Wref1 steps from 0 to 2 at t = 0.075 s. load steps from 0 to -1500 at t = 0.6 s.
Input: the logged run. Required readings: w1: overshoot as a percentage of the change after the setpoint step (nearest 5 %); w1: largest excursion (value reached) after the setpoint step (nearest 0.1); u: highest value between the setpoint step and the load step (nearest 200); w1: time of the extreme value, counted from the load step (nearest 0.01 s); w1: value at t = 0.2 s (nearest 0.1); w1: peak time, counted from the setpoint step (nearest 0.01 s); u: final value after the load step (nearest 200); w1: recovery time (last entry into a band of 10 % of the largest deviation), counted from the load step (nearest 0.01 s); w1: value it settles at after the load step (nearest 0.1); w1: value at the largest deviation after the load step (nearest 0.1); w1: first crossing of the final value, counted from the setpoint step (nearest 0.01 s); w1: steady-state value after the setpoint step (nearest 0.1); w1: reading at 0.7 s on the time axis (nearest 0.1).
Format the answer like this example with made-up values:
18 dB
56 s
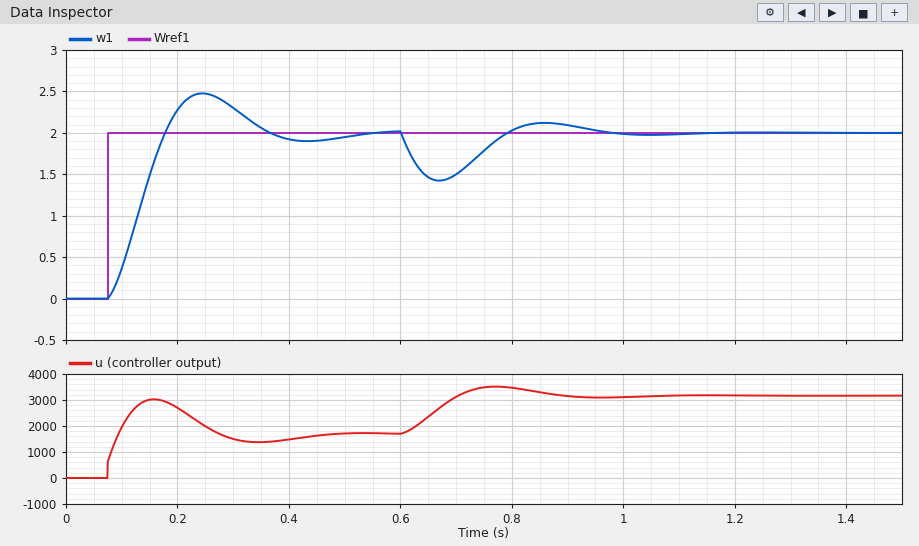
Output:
25 %
2.5
3000
0.07 s
2.3
0.17 s
3200
0.33 s
2.0
1.4
0.10 s
2.0
1.5
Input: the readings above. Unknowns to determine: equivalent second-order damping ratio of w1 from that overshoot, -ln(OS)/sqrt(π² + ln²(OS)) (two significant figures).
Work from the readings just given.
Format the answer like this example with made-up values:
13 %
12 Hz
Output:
0.40
